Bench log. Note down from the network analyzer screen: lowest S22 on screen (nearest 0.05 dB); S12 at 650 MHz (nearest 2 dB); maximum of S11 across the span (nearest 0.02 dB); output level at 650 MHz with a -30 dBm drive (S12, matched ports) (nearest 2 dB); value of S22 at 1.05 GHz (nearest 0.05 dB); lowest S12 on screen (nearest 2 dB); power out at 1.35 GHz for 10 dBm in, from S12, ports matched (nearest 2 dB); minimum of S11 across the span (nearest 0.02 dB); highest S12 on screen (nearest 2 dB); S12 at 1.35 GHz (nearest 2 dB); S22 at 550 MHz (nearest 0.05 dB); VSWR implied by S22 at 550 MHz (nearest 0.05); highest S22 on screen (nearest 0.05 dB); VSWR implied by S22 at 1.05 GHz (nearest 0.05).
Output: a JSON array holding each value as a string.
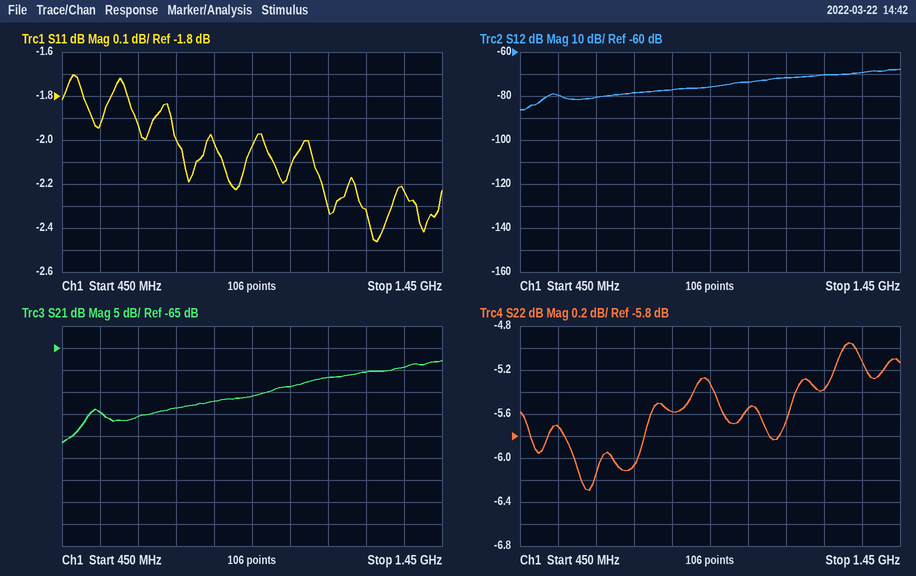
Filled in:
["-6.30 dB", "-80 dB", "-1.70 dB", "-110 dBm", "-5.55 dB", "-86 dB", "-60 dBm", "-2.46 dB", "-68 dB", "-70 dB", "-5.70 dB", "3.15", "-4.95 dB", "3.25"]
